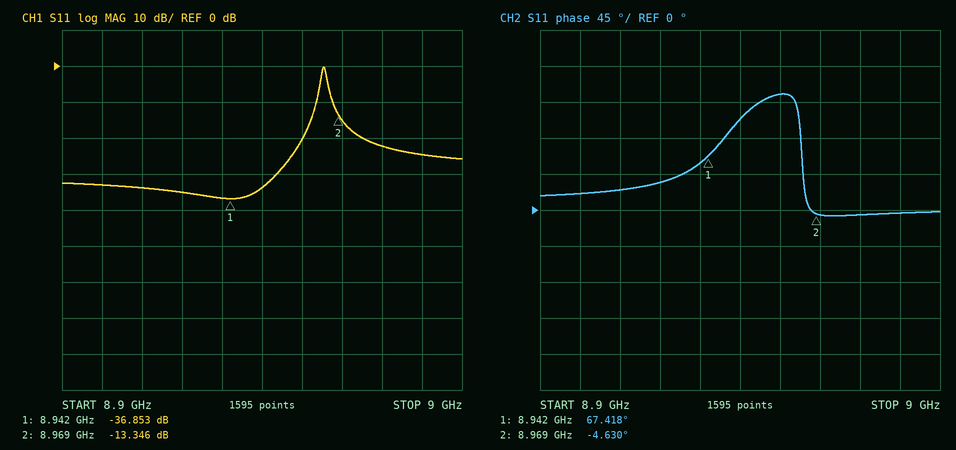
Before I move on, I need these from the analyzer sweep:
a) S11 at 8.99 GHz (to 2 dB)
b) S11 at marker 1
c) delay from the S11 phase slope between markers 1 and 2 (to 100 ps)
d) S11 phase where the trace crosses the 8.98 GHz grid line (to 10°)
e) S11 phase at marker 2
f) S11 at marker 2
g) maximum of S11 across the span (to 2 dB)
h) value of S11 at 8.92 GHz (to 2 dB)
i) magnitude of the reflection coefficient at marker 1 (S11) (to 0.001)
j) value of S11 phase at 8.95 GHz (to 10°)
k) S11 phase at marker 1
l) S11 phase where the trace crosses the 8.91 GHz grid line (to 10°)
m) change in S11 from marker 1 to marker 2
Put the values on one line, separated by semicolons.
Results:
-24 dB; -36.853 dB; 7.4 ns; -10°; -4.630°; -13.346 dB; 0 dB; -34 dB; 0.014; 110°; 67.418°; 20°; 23.507 dB
